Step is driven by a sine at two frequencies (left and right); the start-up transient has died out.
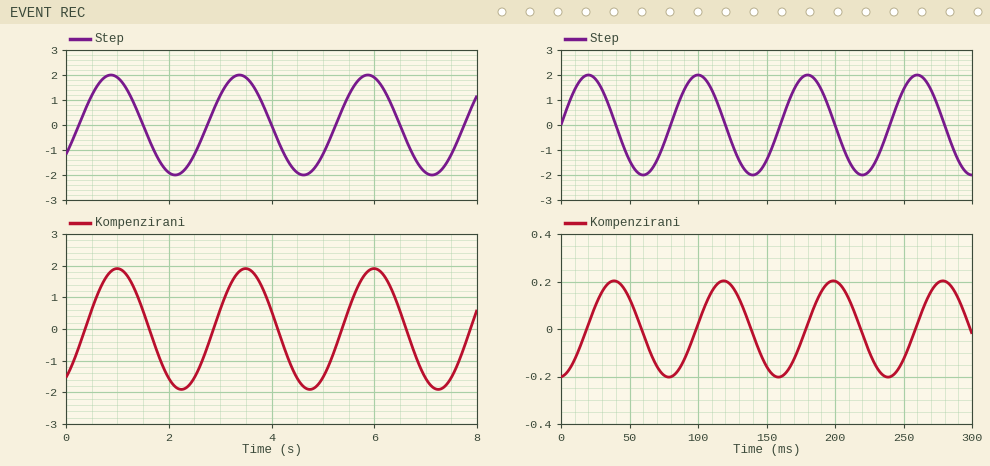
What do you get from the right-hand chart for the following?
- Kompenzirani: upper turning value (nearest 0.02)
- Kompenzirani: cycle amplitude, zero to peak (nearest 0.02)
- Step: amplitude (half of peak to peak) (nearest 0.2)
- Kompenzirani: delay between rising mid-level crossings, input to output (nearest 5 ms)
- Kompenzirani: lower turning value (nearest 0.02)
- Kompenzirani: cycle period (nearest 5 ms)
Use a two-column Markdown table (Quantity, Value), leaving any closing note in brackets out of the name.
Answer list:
| Quantity | Value |
|---|---|
| Kompenzirani: upper turning value | 0.20 |
| Kompenzirani: cycle amplitude, zero to peak | 0.20 |
| Step: amplitude (half of peak to peak) | 2.0 |
| Kompenzirani: delay between rising mid-level crossings, input to output | 20 ms |
| Kompenzirani: lower turning value | -0.20 |
| Kompenzirani: cycle period | 80 ms |
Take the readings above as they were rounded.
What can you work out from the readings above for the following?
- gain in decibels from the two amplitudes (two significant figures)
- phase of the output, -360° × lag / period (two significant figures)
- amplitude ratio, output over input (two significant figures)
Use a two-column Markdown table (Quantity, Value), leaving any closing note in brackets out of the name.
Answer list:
| Quantity | Value |
|---|---|
| gain in decibels from the two amplitudes | -20 dB |
| phase of the output, -360° × lag / period | -90° |
| amplitude ratio, output over input | 0.10 |
